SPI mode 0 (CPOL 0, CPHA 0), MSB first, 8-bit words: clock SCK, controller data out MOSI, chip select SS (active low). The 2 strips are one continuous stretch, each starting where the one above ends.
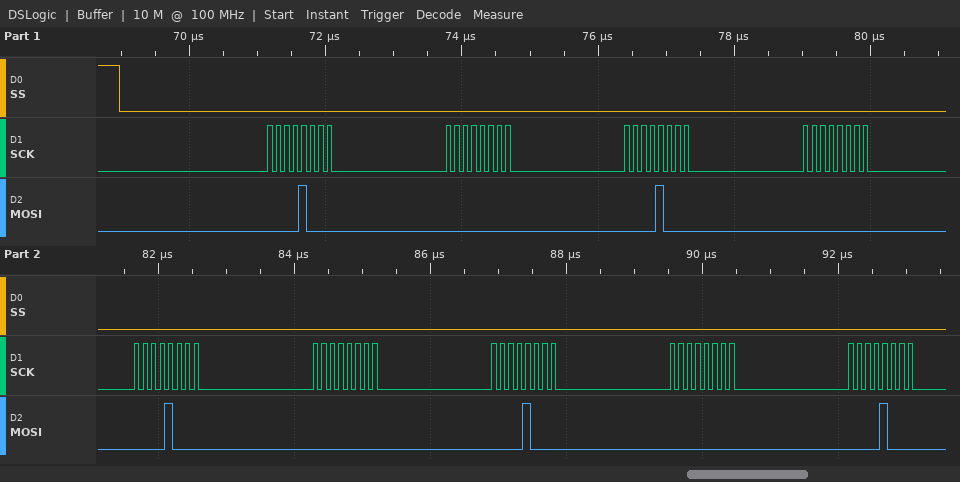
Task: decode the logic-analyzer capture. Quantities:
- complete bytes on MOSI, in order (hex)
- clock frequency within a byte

08 00 08 00 08 00 08 00 08
8 MHz
